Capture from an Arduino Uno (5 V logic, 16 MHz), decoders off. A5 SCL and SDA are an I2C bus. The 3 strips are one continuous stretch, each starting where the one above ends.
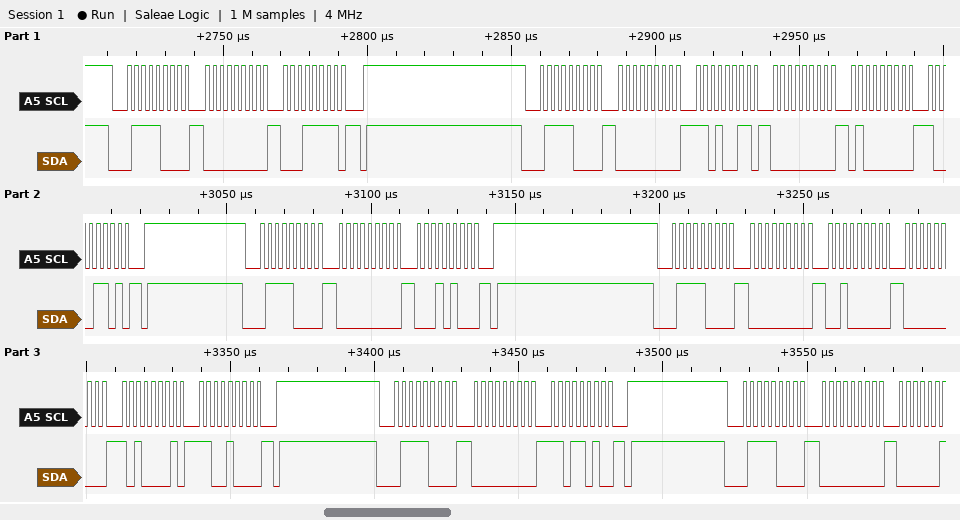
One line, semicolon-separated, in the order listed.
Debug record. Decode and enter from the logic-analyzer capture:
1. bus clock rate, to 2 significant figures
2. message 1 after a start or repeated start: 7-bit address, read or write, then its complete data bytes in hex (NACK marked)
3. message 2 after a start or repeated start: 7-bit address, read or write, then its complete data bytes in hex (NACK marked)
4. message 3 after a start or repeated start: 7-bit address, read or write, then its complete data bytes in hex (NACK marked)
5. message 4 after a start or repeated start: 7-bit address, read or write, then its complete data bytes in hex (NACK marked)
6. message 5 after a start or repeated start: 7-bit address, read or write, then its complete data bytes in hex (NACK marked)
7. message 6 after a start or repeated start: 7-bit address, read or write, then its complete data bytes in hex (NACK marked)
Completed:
400 kHz; 0x3C write: 00 1F; 0x3C write: 00 D3 00 40 8D; 0x3C write: 00 14; 0x3C write: 00 20 00 A1 C8; 0x3C write: 00 DA; 0x3C write: 00
